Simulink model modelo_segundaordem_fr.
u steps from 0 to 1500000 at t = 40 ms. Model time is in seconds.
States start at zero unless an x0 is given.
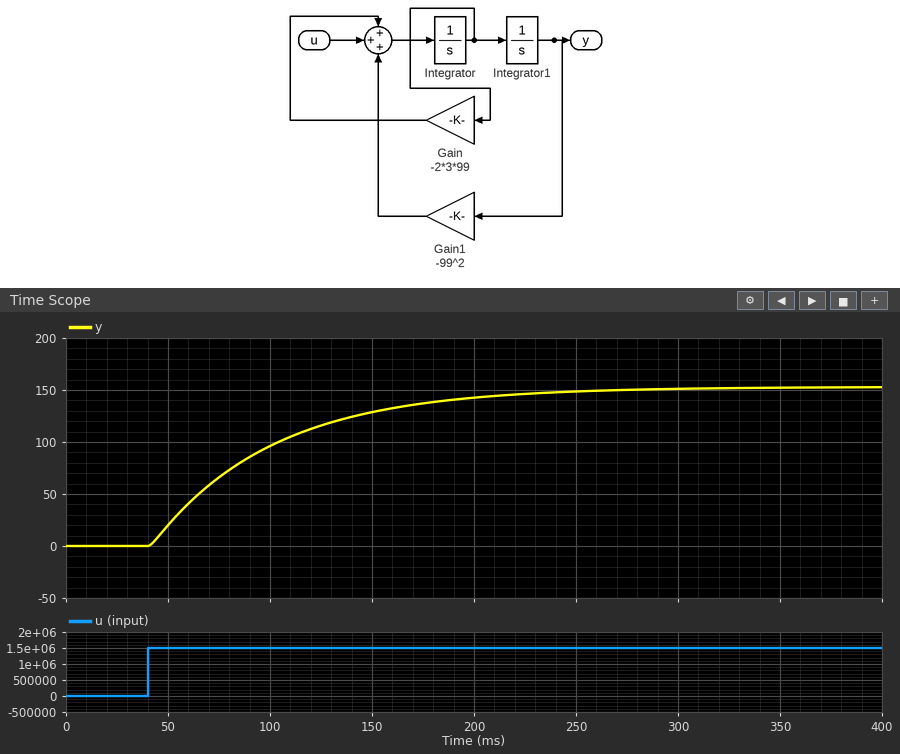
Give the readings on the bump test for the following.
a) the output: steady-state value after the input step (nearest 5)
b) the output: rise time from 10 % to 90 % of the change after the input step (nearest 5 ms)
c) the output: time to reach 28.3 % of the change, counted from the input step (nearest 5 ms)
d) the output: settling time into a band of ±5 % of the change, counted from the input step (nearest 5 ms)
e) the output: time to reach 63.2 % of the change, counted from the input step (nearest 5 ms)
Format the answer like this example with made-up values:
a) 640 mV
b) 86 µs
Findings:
a) 155
b) 130 ms
c) 20 ms
d) 180 ms
e) 60 ms
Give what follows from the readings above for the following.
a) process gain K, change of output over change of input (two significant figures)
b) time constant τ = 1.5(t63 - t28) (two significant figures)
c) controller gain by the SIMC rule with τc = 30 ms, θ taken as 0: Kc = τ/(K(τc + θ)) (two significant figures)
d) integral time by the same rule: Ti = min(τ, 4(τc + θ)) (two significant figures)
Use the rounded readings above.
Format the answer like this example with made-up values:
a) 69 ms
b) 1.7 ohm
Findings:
a) 0.00010
b) 60 ms
c) 20000
d) 60 ms
